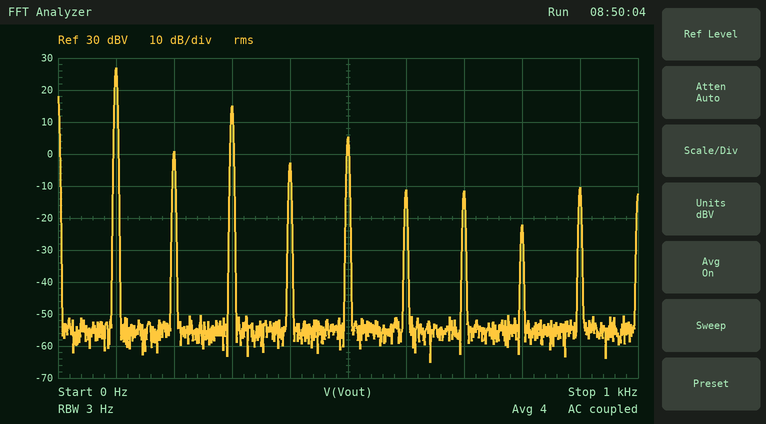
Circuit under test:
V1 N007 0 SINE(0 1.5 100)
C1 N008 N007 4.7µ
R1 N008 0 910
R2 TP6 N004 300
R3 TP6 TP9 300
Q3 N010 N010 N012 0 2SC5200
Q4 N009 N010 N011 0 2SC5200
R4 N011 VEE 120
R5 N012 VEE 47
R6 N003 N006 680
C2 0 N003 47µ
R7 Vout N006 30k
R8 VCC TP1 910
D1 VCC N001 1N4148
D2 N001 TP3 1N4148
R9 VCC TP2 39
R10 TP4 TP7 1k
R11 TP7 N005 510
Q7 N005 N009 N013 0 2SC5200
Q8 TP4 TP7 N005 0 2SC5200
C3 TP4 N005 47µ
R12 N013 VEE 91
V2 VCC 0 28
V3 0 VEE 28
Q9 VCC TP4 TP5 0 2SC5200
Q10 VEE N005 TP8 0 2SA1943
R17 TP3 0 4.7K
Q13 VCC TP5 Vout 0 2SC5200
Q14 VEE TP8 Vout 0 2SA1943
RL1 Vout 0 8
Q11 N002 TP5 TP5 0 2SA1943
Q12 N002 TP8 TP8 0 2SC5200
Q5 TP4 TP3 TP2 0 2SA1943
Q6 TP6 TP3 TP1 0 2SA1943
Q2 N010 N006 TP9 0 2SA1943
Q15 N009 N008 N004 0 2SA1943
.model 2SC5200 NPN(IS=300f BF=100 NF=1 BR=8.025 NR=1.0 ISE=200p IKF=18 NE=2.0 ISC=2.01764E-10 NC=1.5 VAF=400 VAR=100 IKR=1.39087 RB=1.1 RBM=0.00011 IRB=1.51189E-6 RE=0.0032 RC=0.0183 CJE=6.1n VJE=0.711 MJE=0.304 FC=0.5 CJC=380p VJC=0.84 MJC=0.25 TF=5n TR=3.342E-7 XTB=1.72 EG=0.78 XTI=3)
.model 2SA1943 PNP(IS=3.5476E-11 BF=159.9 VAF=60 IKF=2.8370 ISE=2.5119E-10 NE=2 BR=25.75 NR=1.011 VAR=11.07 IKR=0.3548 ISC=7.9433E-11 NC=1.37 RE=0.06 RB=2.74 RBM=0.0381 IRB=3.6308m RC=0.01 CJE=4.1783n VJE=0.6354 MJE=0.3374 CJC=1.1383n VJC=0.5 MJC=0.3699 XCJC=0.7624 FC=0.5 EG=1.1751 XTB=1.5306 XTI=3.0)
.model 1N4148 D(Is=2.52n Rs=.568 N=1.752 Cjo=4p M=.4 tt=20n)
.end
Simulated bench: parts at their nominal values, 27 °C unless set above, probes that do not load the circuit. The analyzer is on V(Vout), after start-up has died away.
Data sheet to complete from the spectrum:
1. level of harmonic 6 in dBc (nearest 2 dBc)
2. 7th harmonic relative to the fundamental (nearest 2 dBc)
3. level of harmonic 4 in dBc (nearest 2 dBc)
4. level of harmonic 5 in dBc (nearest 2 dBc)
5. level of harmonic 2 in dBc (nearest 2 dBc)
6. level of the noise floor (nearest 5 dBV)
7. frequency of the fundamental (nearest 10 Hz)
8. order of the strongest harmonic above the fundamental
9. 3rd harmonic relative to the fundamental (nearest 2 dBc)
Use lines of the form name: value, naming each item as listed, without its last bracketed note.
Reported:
level of harmonic 6 in dBc: -38 dBc
7th harmonic relative to the fundamental: -38 dBc
level of harmonic 4 in dBc: -30 dBc
level of harmonic 5 in dBc: -22 dBc
level of harmonic 2 in dBc: -26 dBc
level of the noise floor: -55 dBV
frequency of the fundamental: 100 Hz
order of the strongest harmonic above the fundamental: 3
3rd harmonic relative to the fundamental: -12 dBc
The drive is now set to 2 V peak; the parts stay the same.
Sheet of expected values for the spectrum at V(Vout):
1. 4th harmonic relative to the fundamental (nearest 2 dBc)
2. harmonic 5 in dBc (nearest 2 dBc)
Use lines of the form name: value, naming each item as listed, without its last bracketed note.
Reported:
4th harmonic relative to the fundamental: -28 dBc
harmonic 5 in dBc: -18 dBc
